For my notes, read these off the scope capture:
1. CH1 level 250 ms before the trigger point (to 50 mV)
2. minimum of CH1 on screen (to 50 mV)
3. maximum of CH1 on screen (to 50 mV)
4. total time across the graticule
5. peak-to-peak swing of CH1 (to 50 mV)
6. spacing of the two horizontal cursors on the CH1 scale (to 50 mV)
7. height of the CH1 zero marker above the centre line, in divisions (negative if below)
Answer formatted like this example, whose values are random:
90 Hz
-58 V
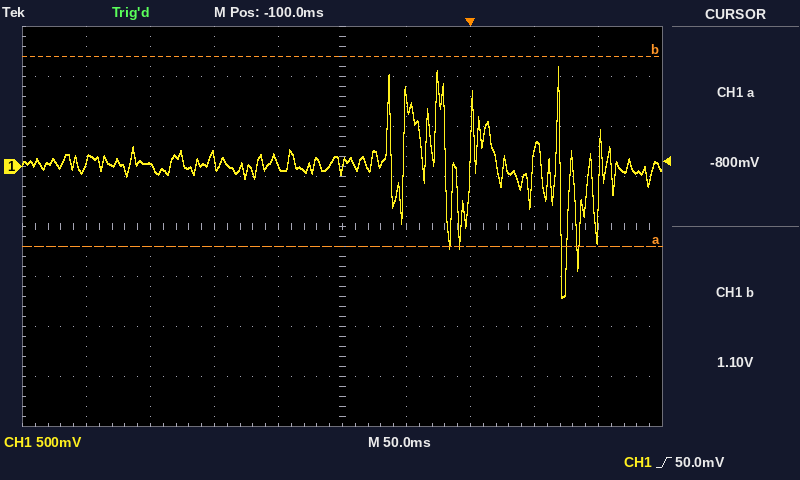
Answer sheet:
0 mV
-1.30 V
1.00 V
500 ms
2.30 V
1.90 V
+1.2 div
